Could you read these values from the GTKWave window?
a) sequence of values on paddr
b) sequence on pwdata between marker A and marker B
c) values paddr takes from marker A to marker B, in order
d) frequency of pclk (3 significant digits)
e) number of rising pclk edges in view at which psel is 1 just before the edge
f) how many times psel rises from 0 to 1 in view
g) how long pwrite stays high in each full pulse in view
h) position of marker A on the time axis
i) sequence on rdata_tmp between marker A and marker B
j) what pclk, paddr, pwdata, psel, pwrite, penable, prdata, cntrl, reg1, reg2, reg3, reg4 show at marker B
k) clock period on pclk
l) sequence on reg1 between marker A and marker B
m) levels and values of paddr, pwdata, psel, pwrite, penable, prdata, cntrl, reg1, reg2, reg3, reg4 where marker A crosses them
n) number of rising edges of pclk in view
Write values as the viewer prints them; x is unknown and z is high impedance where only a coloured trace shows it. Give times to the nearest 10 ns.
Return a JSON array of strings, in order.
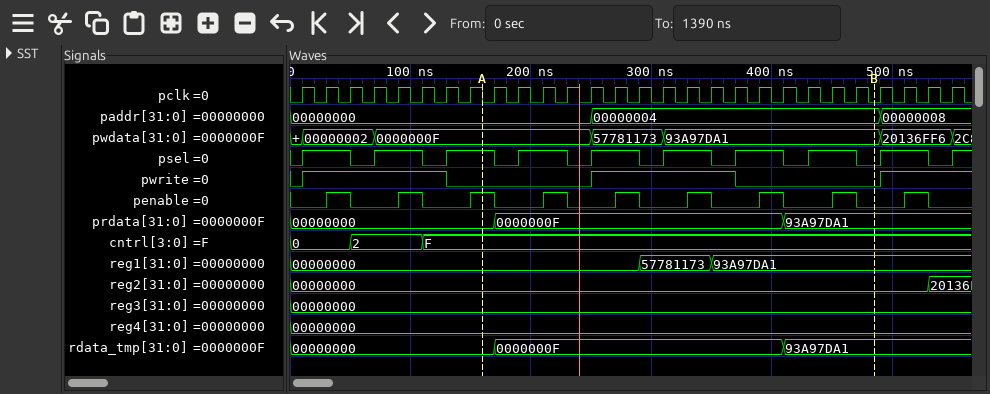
["00000000, 00000004, 00000008", "0000000F, 57781173, 93A97DA1", "00000000, 00000004", "50.0 MHz", "18", "10", "120 ns, 120 ns", "160 ns", "00000000, 0000000F, 93A97DA1", "pclk=0, paddr=00000004, pwdata=93A97DA1, psel=0, pwrite=0, penable=0, prdata=93A97DA1, cntrl=F, reg1=93A97DA1, reg2=00000000, reg3=00000000, reg4=00000000", "20 ns", "00000000, 57781173, 93A97DA1", "paddr=00000000, pwdata=0000000F, psel=1, pwrite=0, penable=1, prdata=00000000, cntrl=F, reg1=00000000, reg2=00000000, reg3=00000000, reg4=00000000", "28"]
